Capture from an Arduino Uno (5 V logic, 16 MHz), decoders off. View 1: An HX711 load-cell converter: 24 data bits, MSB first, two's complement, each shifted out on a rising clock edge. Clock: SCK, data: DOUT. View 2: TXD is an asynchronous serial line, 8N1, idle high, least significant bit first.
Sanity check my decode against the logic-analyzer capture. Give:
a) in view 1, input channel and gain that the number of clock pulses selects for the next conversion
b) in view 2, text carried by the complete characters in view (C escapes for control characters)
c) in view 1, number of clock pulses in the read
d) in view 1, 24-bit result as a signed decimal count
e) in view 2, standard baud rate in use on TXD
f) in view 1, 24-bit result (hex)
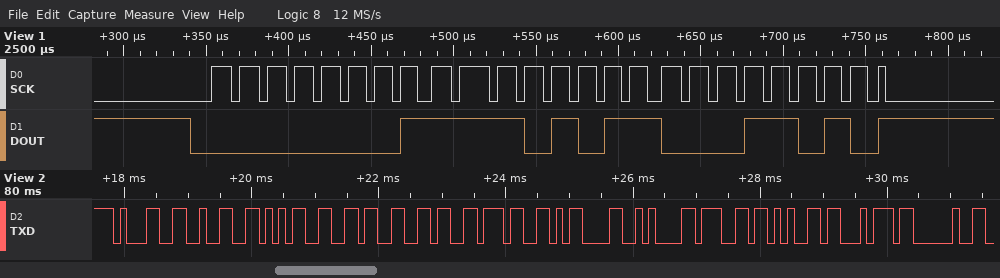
channel A, gain 128
"125667\r\nget "
25
125722
9600 baud
0x01EB1A
